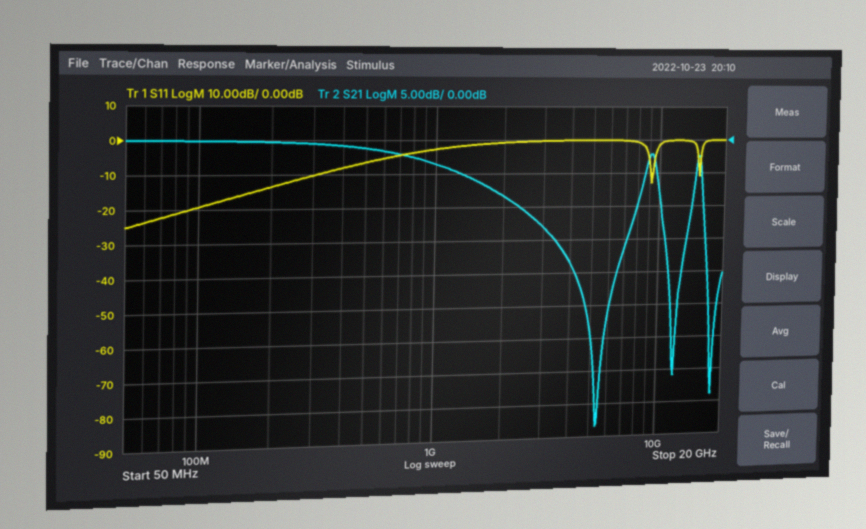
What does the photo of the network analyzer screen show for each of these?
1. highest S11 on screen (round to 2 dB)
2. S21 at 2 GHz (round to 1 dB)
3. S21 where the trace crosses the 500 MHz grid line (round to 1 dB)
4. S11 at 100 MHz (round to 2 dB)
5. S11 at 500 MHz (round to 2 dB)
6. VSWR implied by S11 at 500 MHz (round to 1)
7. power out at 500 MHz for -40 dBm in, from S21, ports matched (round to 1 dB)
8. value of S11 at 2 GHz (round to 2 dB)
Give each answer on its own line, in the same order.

0 dB
-8 dB
-1 dB
-20 dB
-6 dB
3
-41 dBm
0 dB
